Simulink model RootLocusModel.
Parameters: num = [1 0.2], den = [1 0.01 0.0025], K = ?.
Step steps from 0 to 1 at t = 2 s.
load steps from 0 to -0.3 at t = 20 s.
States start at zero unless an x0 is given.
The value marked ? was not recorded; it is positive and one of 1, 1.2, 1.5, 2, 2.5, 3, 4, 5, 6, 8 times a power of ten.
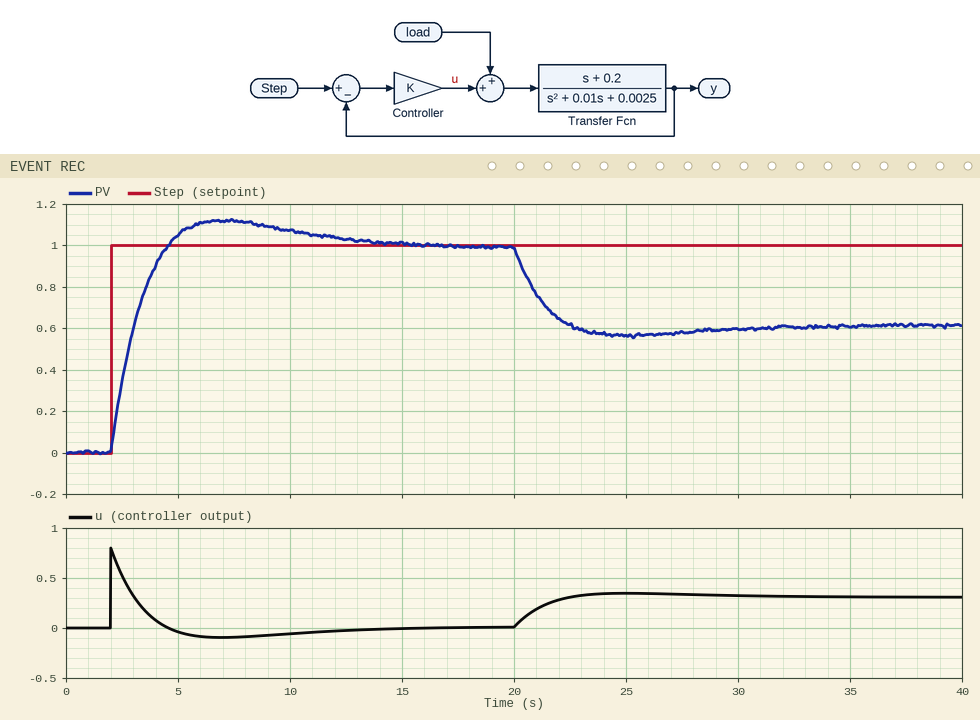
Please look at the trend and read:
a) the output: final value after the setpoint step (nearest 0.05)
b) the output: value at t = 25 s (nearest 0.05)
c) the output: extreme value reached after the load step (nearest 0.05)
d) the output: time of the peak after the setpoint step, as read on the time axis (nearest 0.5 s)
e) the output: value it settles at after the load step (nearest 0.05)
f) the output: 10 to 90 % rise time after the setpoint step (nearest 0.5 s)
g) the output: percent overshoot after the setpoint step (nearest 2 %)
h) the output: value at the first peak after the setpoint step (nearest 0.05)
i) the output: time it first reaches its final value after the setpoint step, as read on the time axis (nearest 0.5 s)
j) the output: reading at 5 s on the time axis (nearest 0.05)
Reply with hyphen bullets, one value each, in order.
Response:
- 1.00
- 0.55
- 0.55
- 7.0 s
- 0.60
- 2.0 s
- 14 %
- 1.10
- 4.5 s
- 1.05
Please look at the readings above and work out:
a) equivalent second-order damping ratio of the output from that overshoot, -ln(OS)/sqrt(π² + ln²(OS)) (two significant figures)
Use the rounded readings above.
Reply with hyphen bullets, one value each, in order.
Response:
- 0.53
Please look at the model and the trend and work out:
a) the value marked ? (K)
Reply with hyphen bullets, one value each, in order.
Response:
- 0.8
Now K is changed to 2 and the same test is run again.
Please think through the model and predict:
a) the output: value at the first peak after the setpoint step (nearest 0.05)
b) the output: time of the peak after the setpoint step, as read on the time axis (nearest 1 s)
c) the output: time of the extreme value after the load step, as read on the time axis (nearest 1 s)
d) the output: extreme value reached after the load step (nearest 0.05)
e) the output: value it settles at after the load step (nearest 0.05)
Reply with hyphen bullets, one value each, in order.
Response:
- 1.05
- 5 s
- 23 s
- 0.85
- 0.85
